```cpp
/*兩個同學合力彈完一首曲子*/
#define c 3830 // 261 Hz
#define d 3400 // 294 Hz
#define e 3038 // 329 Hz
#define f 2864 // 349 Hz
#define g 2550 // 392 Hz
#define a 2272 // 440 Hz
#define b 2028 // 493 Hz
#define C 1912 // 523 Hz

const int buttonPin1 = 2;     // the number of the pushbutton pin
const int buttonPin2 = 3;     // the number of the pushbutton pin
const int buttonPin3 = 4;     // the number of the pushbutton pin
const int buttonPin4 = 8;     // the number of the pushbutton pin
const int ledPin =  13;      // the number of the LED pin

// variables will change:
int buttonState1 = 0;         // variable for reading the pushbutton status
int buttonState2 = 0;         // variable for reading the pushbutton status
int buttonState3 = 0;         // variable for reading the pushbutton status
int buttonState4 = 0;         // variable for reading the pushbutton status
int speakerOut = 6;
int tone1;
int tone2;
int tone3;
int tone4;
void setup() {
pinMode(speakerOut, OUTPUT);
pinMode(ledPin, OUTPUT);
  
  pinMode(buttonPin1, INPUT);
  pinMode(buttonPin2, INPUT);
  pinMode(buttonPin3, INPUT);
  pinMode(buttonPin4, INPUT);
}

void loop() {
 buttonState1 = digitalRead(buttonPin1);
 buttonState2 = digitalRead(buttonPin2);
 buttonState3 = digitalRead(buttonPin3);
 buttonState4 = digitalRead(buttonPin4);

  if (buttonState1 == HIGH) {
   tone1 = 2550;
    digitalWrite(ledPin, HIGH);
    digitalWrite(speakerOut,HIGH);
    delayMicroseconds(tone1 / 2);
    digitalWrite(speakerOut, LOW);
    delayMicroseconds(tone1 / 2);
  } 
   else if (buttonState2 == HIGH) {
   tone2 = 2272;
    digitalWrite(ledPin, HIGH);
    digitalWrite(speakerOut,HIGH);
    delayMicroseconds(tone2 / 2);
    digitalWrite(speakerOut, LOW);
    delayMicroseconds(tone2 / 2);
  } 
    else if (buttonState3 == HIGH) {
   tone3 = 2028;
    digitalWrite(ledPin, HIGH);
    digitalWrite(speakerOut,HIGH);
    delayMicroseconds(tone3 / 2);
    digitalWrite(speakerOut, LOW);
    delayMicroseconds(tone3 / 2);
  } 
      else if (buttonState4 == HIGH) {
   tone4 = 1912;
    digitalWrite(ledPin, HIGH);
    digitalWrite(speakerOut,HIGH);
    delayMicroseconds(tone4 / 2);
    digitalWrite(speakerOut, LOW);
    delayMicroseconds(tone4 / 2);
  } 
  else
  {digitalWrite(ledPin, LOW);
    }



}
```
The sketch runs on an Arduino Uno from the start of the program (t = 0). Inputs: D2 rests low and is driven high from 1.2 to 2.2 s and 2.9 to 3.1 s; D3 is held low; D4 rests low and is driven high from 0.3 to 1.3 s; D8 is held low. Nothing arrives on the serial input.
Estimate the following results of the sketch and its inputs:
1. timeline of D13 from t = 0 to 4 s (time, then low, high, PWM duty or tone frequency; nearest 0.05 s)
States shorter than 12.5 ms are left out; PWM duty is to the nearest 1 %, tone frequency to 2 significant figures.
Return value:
0 s low; 0.3 s high; 2.2 s low; 2.9 s high; 3.1 s low
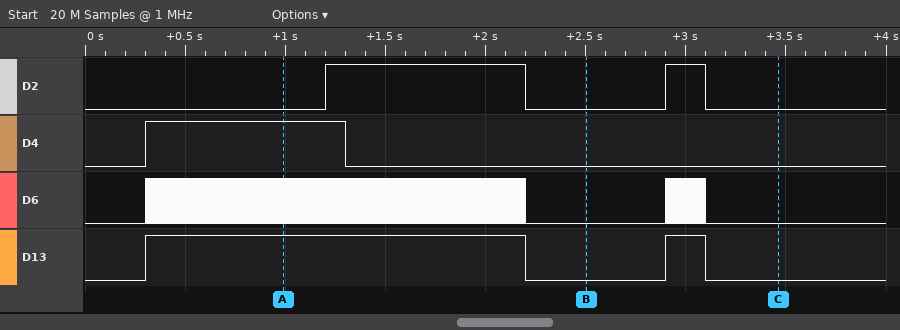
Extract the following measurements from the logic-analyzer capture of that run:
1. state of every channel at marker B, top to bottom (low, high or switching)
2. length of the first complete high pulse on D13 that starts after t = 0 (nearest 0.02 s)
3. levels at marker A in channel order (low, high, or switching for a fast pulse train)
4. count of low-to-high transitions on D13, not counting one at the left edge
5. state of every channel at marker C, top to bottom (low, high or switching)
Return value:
D2 low, D4 low, D6 low, D13 low
1.90 s
D2 low, D4 high, D6 switching, D13 high
2
D2 low, D4 low, D6 low, D13 low
